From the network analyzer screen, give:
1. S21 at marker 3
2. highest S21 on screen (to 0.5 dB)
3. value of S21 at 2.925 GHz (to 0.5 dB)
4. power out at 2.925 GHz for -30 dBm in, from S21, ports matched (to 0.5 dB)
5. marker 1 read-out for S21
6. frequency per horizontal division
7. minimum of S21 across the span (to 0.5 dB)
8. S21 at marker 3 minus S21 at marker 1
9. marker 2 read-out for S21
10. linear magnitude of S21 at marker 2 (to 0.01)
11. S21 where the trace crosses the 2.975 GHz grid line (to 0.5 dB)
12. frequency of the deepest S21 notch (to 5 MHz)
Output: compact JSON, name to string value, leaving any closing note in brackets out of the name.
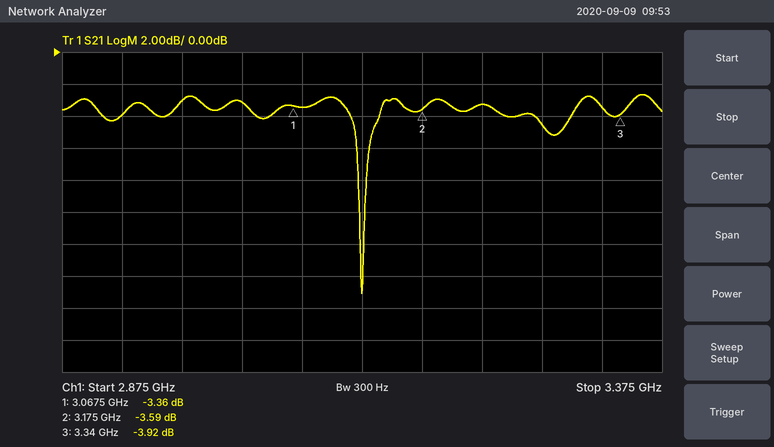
{"S21 at marker 3": "-3.92 dB", "highest S21 on screen": "-2.5 dB", "value of S21 at 2.925 GHz": "-4.0 dB", "power out at 2.925 GHz for -30 dBm in, from S21, ports matched": "-34.0 dBm", "marker 1 read-out for S21": "-3.36 dB", "frequency per horizontal division": "50 MHz", "minimum of S21 across the span": "-15.0 dB", "S21 at marker 3 minus S21 at marker 1": "-0.56 dB", "marker 2 read-out for S21": "-3.59 dB", "linear magnitude of S21 at marker 2": "0.66", "S21 where the trace crosses the 2.975 GHz grid line": "-3.0 dB", "frequency of the deepest S21 notch": "3.125 GHz"}
